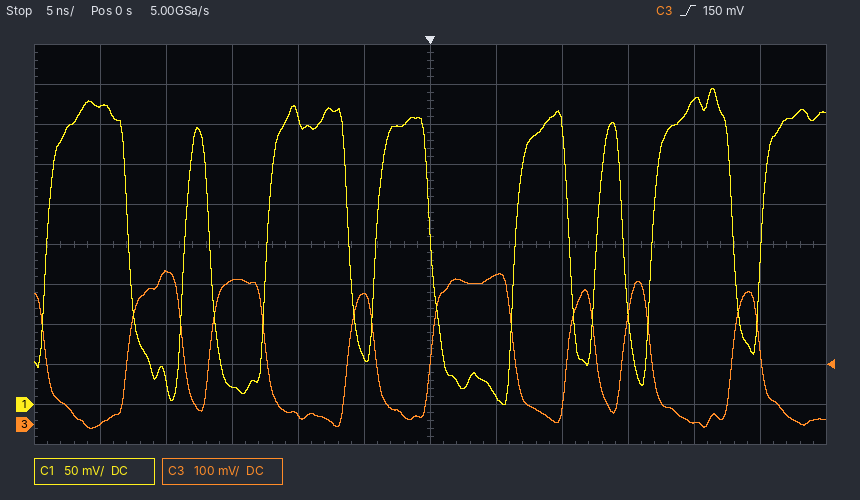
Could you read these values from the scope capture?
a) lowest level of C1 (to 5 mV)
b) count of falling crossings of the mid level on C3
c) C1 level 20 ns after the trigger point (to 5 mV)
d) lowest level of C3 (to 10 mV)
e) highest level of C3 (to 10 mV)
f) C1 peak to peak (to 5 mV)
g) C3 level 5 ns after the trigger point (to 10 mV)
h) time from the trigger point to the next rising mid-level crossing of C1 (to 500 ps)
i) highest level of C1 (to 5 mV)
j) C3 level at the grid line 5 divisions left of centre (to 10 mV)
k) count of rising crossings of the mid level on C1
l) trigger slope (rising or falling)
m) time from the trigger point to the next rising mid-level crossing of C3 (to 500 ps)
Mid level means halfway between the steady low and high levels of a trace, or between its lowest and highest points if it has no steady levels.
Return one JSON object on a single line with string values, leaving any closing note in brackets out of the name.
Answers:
{"lowest level of C1": "0 mV", "count of falling crossings of the mid level on C3": "8", "C1 level 20 ns after the trigger point": "380 mV", "lowest level of C3": "-10 mV", "highest level of C3": "380 mV", "C1 peak to peak": "395 mV", "C3 level 5 ns after the trigger point": "370 mV", "time from the trigger point to the next rising mid-level crossing of C1": "6.5 ns", "highest level of C1": "395 mV", "C3 level at the grid line 5 divisions left of centre": "0 mV", "count of rising crossings of the mid level on C1": "8", "trigger slope": "rising", "time from the trigger point to the next rising mid-level crossing of C3": "10.5 ns"}
